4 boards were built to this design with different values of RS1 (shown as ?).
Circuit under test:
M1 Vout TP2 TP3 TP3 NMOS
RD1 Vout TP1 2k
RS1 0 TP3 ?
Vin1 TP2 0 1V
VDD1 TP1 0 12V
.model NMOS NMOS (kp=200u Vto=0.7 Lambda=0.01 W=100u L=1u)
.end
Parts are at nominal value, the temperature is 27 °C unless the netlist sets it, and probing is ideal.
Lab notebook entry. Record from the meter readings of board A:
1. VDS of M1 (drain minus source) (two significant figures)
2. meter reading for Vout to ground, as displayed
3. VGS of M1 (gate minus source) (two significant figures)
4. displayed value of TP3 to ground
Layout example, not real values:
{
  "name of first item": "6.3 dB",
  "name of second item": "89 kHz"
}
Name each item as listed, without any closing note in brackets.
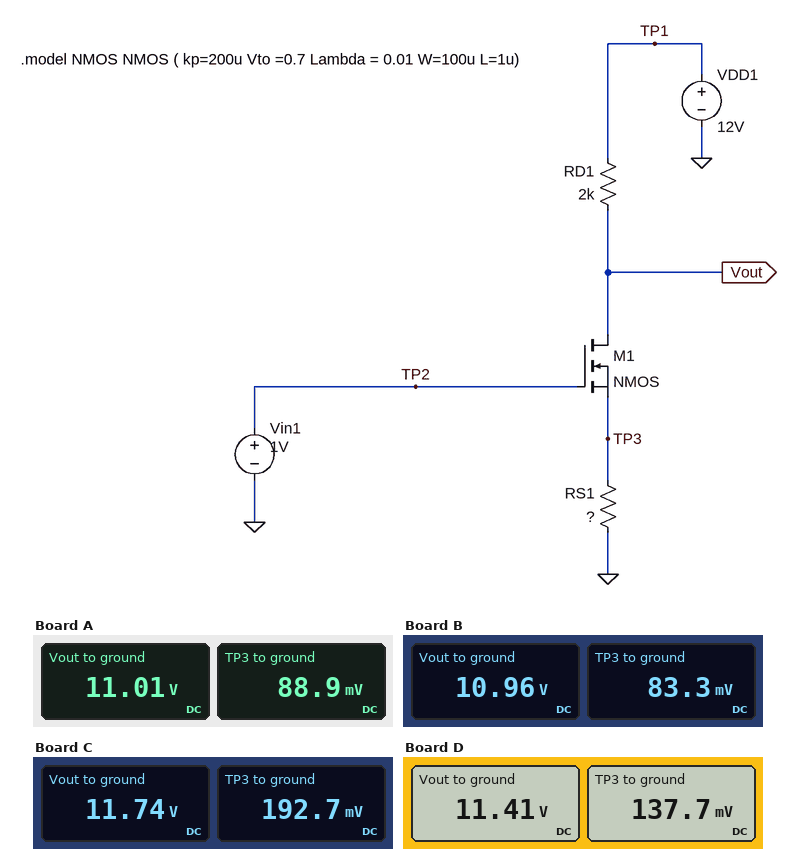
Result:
{
  "VDS of M1 (drain minus source)": "11 V",
  "meter reading for Vout to ground, as displayed": "11.01 V",
  "VGS of M1 (gate minus source)": "910 mV",
  "displayed value of TP3 to ground": "88.9 mV"
}
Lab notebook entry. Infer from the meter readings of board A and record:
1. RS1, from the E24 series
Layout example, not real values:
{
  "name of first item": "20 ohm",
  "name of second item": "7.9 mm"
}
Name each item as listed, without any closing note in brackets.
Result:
{
  "RS1, from the E24 series": "180 Ω"
}
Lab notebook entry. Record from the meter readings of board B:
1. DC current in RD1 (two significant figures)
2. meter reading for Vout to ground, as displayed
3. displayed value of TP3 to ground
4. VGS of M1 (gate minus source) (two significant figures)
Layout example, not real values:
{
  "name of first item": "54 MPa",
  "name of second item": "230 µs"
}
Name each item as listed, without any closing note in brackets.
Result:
{
  "DC current in RD1": "520 µA",
  "meter reading for Vout to ground, as displayed": "10.96 V",
  "displayed value of TP3 to ground": "83.3 mV",
  "VGS of M1 (gate minus source)": "920 mV"
}
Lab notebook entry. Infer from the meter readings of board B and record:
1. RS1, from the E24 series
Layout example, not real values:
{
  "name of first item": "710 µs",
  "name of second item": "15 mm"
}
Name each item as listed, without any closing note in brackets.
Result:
{
  "RS1, from the E24 series": "160 Ω"
}
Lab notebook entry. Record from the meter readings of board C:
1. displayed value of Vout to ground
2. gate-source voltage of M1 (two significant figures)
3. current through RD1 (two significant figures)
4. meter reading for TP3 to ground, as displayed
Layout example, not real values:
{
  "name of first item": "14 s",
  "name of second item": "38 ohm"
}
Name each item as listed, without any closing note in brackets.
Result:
{
  "displayed value of Vout to ground": "11.74 V",
  "gate-source voltage of M1": "810 mV",
  "current through RD1": "130 µA",
  "meter reading for TP3 to ground, as displayed": "192.7 mV"
}
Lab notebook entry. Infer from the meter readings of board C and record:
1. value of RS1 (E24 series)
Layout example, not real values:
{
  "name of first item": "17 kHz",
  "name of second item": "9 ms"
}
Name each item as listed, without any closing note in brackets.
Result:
{
  "value of RS1": "1.5 kΩ"
}
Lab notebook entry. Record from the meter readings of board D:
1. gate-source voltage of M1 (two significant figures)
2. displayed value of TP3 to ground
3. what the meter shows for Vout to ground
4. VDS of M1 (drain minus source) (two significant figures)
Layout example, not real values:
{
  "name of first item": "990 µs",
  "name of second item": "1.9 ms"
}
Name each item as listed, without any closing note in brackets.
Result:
{
  "gate-source voltage of M1": "860 mV",
  "displayed value of TP3 to ground": "137.7 mV",
  "what the meter shows for Vout to ground": "11.41 V",
  "VDS of M1 (drain minus source)": "11 V"
}
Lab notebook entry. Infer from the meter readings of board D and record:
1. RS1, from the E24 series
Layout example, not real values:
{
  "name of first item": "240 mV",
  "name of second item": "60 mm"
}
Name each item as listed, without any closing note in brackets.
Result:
{
  "RS1, from the E24 series": "470 Ω"
}
